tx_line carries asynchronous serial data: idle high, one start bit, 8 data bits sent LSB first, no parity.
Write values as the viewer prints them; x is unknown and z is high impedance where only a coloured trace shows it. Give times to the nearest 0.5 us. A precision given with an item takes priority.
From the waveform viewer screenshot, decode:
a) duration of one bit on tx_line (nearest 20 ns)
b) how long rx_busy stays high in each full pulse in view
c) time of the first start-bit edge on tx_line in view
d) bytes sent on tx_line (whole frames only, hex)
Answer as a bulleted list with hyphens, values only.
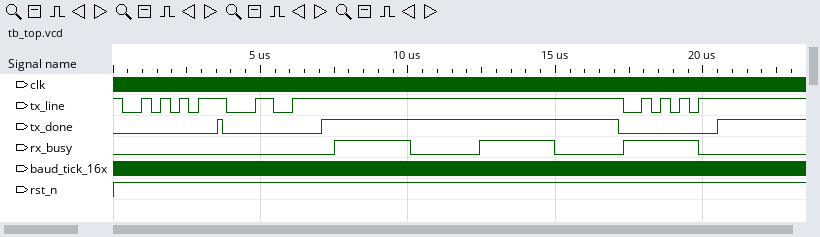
- 320 ns
- 2.5 us, 2.5 us, 2.5 us
- 0.5 us
- AA, CC, AA
